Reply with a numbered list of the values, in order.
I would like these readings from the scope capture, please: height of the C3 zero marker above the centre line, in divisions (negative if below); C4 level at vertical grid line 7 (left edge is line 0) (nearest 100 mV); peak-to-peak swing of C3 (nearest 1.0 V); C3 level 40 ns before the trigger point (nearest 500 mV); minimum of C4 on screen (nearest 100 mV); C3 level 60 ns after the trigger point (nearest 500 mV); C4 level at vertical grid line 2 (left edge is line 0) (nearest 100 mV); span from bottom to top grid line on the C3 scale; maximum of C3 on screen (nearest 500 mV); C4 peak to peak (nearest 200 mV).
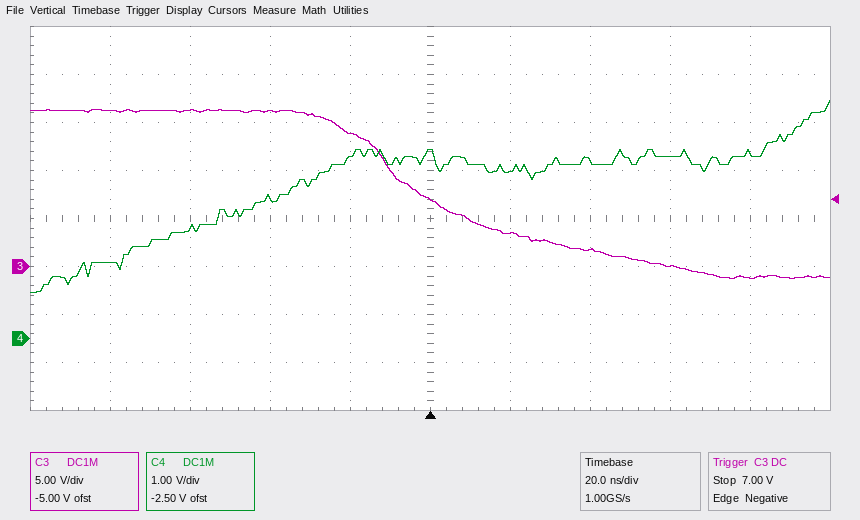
1. -1.0 div
2. 3.7 V
3. 18.0 V
4. 16.0 V
5. 1.0 V
6. 0.0 V
7. 2.3 V
8. 40 V
9. 16.5 V
10. 4.0 V
